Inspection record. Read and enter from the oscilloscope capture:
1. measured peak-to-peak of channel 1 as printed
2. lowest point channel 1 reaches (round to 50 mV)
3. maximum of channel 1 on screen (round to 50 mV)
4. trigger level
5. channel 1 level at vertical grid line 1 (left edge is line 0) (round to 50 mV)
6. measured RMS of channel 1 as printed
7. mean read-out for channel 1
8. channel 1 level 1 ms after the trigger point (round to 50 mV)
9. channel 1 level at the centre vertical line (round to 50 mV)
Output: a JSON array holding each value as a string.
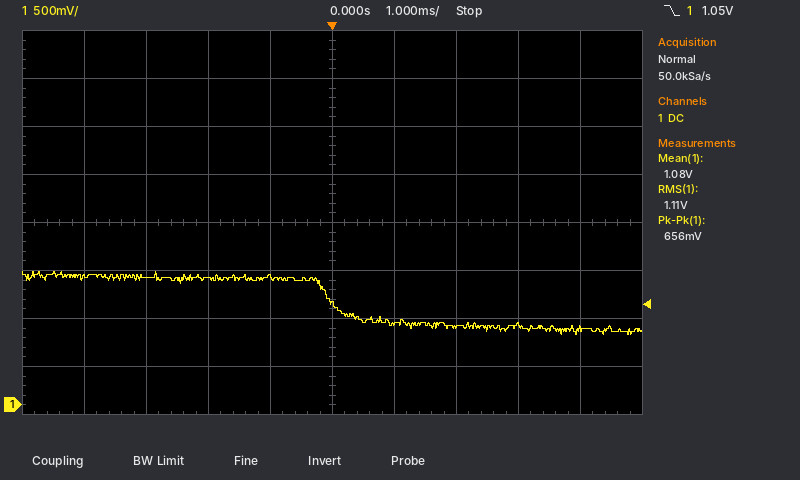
["656 mV", "750 mV", "1.40 V", "1.05 V", "1.35 V", "1.11 V", "1.08 V", "850 mV", "1.05 V"]
